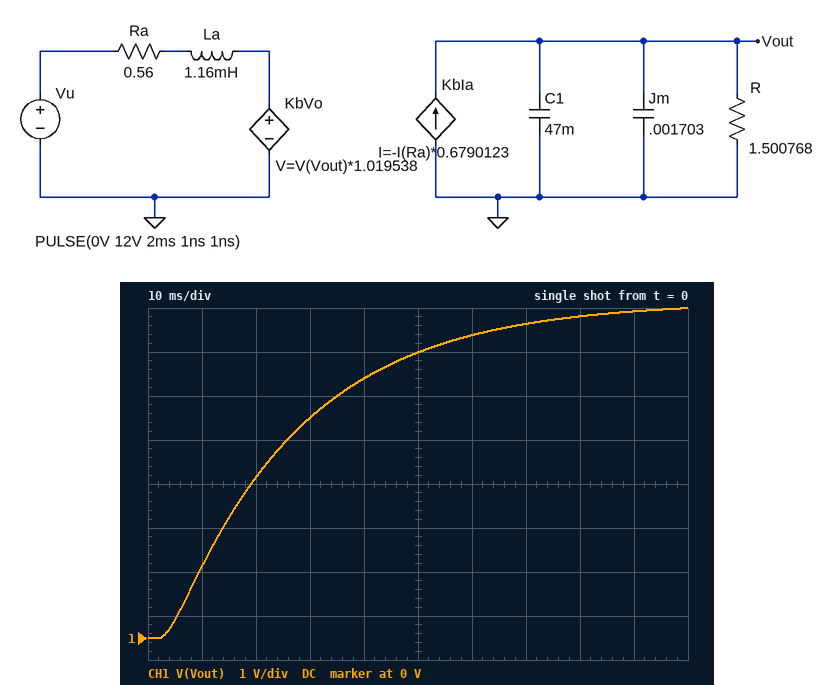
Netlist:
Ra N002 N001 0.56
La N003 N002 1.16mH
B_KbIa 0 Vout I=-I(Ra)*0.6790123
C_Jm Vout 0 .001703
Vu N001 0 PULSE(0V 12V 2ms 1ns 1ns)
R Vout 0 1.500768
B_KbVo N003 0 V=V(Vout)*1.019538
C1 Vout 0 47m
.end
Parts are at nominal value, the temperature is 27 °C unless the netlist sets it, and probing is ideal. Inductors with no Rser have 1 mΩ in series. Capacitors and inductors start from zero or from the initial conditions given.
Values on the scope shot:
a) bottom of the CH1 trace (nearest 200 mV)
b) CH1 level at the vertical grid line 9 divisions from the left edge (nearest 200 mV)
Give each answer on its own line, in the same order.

0 V
7.4 V
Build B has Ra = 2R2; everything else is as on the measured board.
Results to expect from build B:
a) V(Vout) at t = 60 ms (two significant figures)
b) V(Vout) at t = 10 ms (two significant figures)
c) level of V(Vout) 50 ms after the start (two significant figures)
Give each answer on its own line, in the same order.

2.6 V
530 mV
2.3 V
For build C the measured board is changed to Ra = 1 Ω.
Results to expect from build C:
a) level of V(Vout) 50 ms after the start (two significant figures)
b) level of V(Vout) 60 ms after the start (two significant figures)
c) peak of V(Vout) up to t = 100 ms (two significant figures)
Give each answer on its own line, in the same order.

4.4 V
4.8 V
5.6 V
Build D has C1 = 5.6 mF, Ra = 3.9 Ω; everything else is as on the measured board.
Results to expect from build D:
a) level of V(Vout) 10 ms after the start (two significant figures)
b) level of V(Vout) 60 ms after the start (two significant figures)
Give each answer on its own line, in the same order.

1.5 V
2.5 V
